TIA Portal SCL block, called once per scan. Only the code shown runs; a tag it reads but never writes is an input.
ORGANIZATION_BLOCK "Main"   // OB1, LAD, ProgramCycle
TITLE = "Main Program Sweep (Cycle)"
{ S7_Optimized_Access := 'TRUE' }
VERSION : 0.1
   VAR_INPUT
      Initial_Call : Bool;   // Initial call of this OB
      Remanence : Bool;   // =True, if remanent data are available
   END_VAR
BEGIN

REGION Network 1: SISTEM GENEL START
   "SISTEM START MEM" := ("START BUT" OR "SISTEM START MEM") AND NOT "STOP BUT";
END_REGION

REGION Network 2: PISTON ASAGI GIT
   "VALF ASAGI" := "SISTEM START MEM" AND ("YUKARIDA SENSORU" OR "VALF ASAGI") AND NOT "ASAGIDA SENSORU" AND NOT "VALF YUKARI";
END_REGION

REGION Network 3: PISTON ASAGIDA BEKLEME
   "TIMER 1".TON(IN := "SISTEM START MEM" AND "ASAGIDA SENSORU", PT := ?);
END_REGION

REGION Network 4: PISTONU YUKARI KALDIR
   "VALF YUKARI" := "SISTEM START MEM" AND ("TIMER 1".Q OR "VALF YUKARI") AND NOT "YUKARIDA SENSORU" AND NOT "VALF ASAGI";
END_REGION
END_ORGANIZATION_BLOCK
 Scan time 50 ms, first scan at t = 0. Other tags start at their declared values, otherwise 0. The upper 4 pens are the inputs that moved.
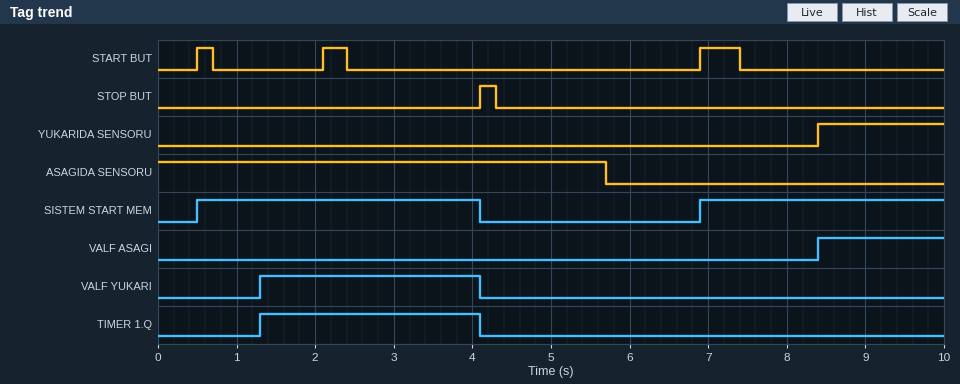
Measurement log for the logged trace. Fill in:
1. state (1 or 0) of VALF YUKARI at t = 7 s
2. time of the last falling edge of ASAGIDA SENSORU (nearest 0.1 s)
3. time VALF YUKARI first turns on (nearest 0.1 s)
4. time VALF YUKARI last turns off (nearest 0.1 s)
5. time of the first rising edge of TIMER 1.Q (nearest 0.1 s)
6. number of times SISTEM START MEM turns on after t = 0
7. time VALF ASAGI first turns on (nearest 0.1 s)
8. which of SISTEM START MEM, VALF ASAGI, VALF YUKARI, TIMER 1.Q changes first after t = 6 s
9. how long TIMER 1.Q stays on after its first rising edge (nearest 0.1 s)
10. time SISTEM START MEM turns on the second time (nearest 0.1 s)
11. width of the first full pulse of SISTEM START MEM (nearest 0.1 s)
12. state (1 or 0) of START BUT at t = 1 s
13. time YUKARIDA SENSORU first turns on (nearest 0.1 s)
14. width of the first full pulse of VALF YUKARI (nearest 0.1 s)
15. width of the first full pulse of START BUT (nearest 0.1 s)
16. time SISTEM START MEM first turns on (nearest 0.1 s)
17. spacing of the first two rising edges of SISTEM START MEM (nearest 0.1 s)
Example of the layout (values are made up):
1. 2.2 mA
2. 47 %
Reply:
1. 0
2. 5.7 s
3. 1.3 s
4. 4.1 s
5. 1.3 s
6. 2
7. 8.4 s
8. SISTEM START MEM
9. 2.8 s
10. 6.9 s
11. 3.6 s
12. 0
13. 8.4 s
14. 2.8 s
15. 0.2 s
16. 0.5 s
17. 6.4 s
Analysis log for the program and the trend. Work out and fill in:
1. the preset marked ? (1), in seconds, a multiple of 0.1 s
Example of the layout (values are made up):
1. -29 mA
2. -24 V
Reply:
1. 0.8 s
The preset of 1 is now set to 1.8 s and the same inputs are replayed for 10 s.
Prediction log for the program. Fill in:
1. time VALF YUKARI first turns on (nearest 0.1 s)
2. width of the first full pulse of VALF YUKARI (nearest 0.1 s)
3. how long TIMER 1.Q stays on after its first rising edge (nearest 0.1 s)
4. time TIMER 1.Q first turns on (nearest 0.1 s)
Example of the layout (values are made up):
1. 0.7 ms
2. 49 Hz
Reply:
1. 2.3 s
2. 1.8 s
3. 1.8 s
4. 2.3 s
